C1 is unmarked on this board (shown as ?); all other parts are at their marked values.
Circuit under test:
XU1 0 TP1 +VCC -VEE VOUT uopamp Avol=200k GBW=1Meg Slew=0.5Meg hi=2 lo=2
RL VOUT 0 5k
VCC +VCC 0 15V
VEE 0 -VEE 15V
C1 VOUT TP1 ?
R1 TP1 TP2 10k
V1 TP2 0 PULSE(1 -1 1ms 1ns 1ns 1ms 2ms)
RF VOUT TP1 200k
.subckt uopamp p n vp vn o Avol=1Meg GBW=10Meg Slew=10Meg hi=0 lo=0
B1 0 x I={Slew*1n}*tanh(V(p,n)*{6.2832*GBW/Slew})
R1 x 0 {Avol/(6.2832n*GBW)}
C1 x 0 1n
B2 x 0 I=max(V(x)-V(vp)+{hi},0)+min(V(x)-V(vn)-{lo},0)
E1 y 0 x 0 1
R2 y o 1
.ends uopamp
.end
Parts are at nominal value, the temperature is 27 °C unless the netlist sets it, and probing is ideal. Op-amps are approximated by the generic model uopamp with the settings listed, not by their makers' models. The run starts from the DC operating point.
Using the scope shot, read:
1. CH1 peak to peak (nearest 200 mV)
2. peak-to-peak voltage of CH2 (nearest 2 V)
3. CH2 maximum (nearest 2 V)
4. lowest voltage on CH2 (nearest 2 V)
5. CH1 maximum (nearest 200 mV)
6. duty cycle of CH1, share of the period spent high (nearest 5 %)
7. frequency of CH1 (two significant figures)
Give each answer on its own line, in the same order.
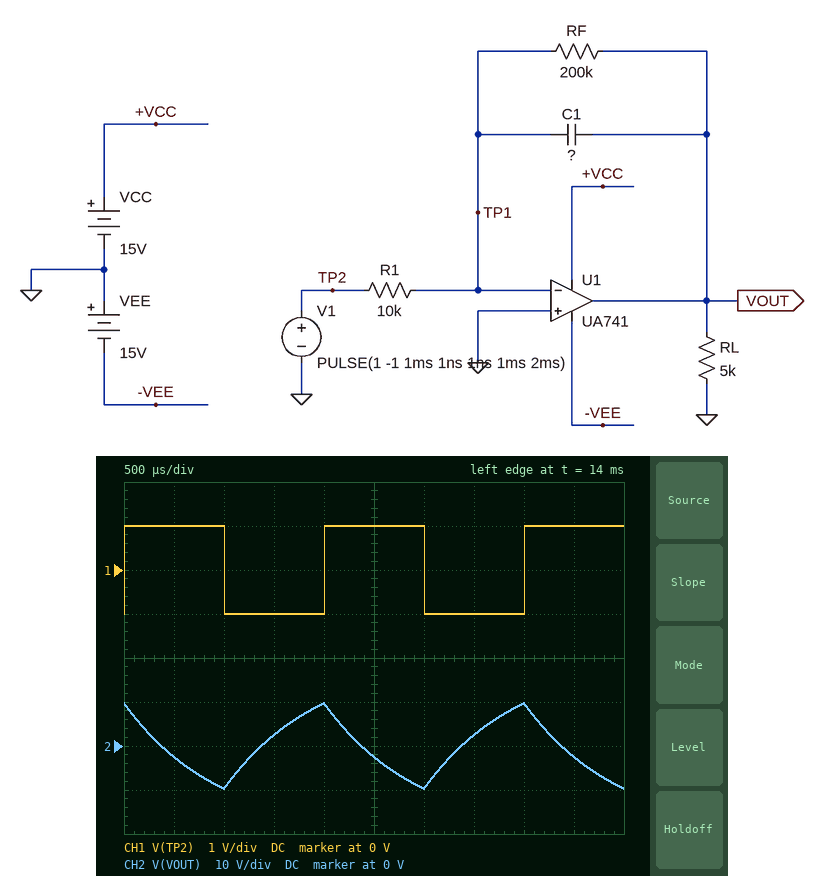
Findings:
2.0 V
20 V
10 V
-10 V
1.0 V
50 %
500 Hz
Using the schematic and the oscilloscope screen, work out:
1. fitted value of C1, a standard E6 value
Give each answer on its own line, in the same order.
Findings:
4.7 nF
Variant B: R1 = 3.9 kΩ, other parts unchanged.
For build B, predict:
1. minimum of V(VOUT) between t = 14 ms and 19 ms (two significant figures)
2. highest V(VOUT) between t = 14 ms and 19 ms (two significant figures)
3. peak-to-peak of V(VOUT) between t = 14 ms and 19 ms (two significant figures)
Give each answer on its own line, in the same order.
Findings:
-13 V
13 V
26 V
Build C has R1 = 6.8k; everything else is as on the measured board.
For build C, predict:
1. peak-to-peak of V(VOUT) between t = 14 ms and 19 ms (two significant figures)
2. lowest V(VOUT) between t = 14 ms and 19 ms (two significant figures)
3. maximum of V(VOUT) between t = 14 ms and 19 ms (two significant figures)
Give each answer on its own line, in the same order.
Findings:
26 V
-13 V
13 V
